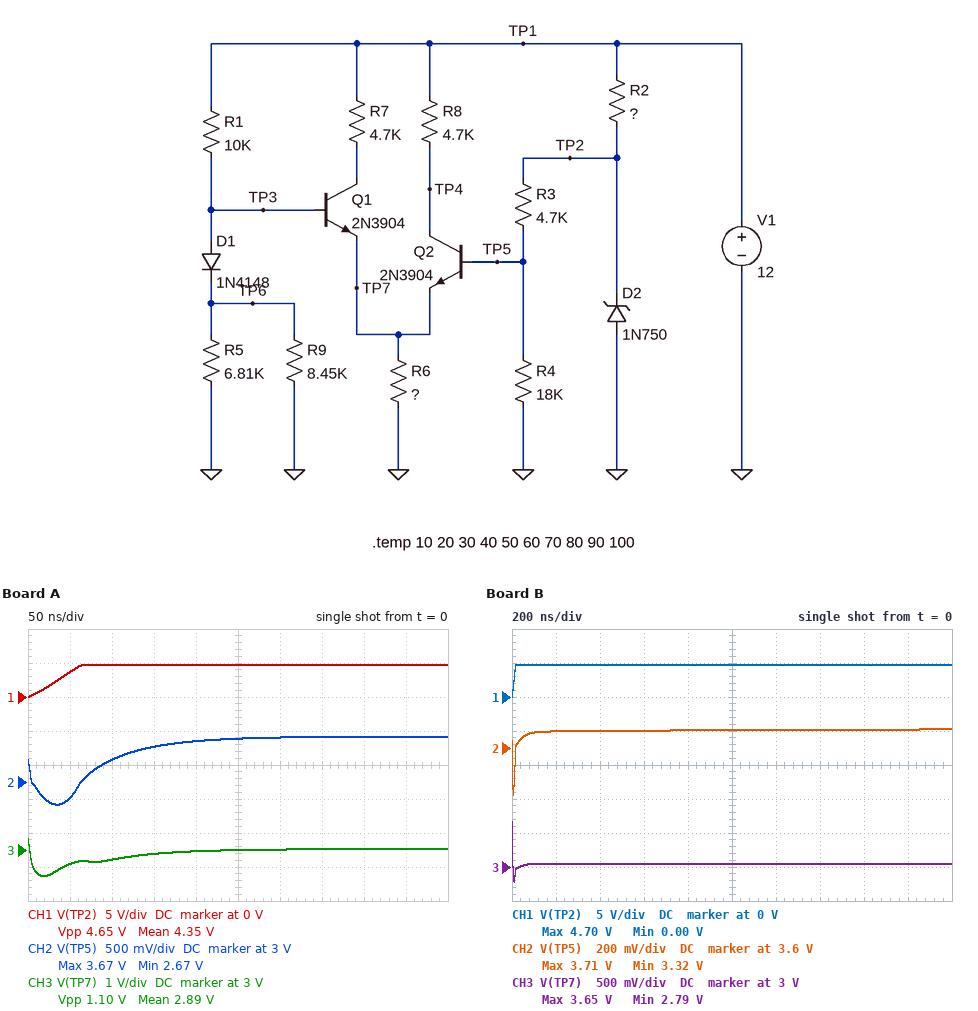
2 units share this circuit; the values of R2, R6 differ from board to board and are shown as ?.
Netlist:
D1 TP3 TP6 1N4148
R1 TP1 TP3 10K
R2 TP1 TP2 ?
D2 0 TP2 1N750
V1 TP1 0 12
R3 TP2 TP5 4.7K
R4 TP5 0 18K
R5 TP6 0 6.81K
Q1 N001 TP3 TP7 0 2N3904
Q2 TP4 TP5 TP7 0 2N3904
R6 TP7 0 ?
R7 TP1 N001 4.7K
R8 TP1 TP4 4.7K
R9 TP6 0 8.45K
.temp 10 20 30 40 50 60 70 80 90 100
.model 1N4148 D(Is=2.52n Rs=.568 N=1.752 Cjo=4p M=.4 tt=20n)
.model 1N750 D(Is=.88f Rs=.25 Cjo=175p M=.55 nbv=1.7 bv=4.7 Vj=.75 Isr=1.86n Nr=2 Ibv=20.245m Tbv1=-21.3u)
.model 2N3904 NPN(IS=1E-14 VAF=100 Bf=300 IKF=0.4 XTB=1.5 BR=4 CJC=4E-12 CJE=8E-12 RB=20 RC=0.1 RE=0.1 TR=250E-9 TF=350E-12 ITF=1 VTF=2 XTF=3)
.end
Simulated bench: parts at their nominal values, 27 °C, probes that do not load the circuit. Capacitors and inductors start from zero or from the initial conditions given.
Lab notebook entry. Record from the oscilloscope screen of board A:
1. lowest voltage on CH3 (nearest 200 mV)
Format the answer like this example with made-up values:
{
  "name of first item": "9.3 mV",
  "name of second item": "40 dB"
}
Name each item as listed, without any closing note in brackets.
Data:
{
  "lowest voltage on CH3": "2.2 V"
}
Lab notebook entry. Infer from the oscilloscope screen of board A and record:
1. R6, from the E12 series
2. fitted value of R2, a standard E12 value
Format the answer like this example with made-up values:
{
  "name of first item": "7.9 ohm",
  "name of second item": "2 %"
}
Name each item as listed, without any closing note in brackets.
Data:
{
  "R6, from the E12 series": "1.2 kΩ",
  "fitted value of R2, a standard E12 value": "1.5 kΩ"
}
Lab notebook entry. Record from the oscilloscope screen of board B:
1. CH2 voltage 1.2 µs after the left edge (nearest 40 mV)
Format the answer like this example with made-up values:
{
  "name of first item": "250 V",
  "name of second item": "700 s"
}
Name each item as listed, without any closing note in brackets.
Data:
{
  "CH2 voltage 1.2 µs after the left edge": "3.72 V"
}
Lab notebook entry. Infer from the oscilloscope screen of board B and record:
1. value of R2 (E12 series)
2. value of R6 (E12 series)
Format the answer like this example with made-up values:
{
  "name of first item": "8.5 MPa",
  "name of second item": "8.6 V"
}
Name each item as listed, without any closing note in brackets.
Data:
{
  "value of R2": "390 Ω",
  "value of R6": "1.5 kΩ"
}
